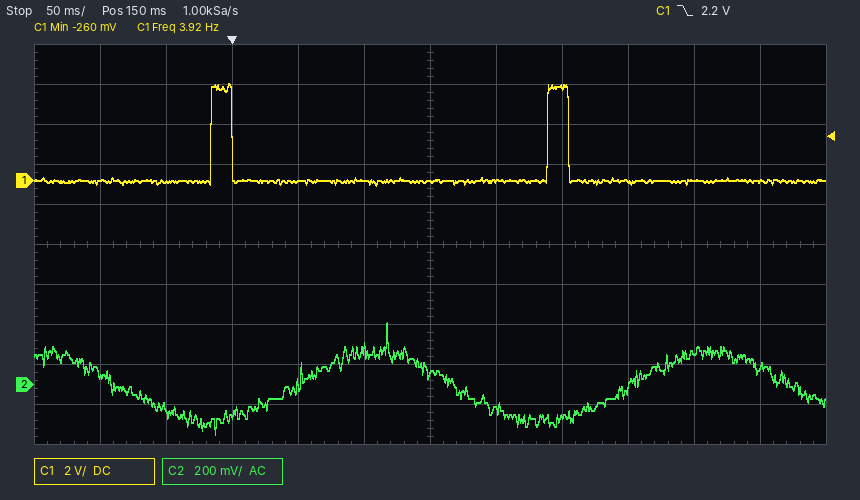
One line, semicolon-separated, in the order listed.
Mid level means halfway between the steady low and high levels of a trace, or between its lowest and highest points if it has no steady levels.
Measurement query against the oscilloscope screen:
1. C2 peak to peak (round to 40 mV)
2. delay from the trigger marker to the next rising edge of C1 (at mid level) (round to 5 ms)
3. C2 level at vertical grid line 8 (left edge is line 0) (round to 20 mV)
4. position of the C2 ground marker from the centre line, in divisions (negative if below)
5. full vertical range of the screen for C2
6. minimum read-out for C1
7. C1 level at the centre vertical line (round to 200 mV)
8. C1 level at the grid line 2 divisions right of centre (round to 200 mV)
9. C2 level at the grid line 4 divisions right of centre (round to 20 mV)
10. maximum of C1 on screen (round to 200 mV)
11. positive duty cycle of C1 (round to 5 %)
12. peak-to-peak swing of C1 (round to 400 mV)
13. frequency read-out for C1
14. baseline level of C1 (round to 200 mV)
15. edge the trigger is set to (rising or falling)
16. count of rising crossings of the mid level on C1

560 mV; 240 ms; -160 mV; -3.5 div; 2 V; -260 mV; 0.0 V; 4.6 V; 160 mV; 4.8 V; 5 %; 5.2 V; 3.92 Hz; 0.0 V; falling; 2
